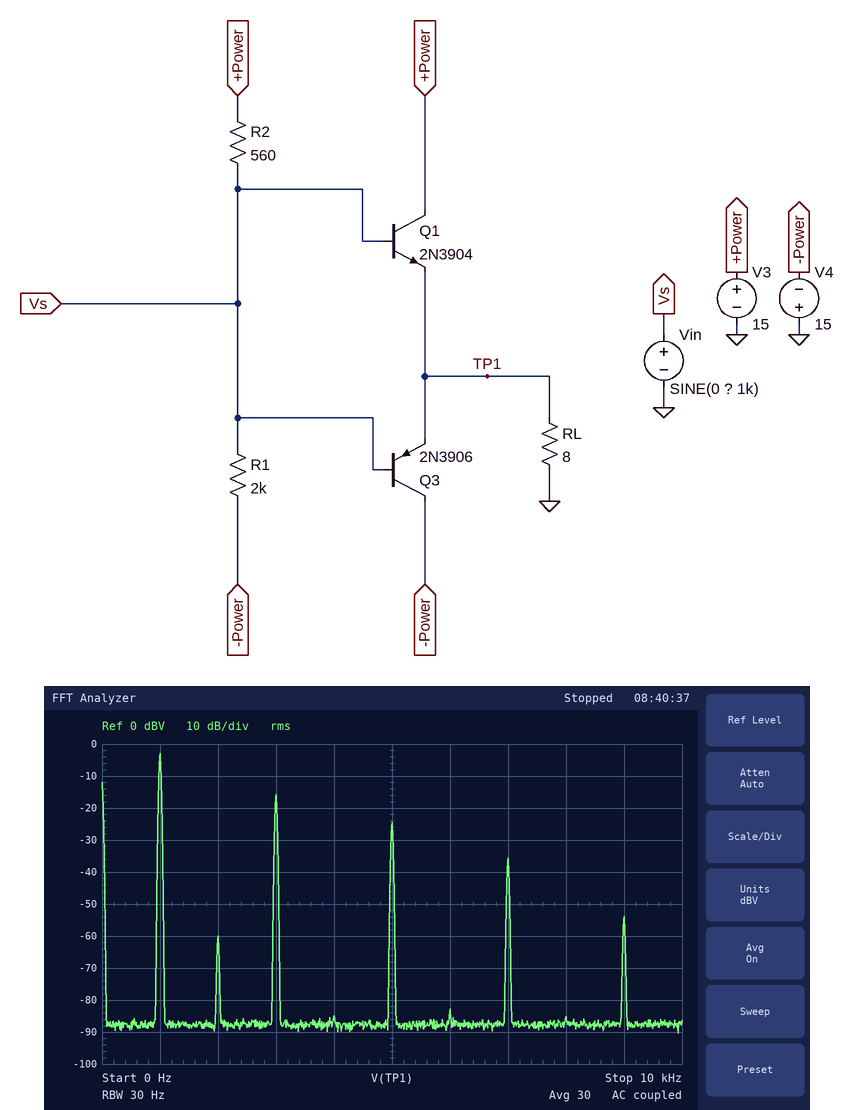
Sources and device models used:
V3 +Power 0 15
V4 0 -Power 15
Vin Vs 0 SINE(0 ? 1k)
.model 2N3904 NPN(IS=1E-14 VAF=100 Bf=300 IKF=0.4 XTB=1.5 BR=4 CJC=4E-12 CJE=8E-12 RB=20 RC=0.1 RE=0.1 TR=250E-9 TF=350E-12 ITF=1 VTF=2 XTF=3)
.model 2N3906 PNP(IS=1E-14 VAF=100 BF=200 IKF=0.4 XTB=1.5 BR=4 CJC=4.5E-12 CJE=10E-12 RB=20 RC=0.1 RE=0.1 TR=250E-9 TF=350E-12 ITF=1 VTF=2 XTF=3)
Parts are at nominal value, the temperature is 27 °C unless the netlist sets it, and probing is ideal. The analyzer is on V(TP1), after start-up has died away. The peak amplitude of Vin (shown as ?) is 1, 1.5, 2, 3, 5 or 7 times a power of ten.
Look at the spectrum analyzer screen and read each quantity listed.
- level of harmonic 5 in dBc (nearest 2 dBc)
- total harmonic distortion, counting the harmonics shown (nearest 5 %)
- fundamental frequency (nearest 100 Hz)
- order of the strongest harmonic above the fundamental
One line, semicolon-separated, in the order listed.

-22 dBc; 25 %; 1.0 kHz; 3
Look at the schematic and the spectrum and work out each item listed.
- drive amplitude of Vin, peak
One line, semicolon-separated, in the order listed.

2 V
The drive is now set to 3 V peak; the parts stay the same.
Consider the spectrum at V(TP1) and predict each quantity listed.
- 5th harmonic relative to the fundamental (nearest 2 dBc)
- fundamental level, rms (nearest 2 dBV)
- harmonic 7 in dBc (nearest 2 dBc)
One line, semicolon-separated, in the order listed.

-24 dBc; 2 dBV; -30 dBc
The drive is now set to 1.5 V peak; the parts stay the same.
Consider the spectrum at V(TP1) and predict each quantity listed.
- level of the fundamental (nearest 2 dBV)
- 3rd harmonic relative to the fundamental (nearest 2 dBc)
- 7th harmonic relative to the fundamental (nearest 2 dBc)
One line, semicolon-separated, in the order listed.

-8 dBV; -10 dBc; -38 dBc
